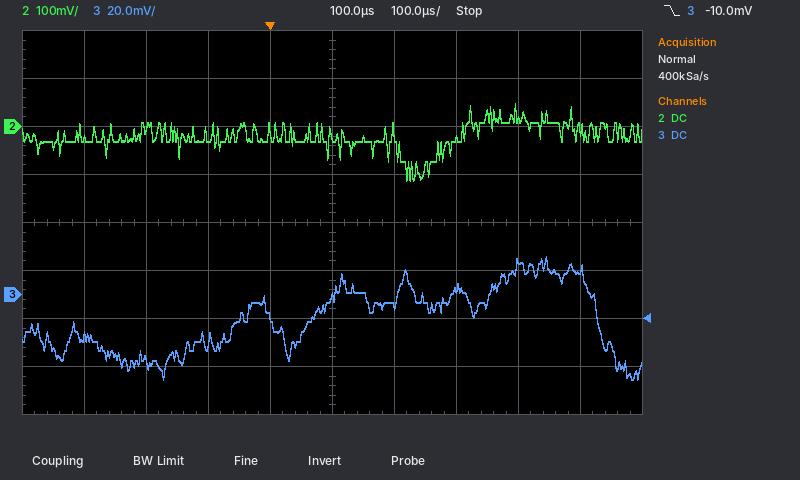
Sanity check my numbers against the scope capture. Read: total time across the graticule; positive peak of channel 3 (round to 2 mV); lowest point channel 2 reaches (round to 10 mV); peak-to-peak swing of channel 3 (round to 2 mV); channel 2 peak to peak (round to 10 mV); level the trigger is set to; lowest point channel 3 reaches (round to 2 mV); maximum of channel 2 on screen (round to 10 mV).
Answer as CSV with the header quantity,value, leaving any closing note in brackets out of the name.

quantity,value
total time across the graticule,1 ms
positive peak of channel 3,16 mV
lowest point channel 2 reaches,-110 mV
peak-to-peak swing of channel 3,52 mV
channel 2 peak to peak,160 mV
level the trigger is set to,-10.0 mV
lowest point channel 3 reaches,-36 mV
maximum of channel 2 on screen,50 mV
